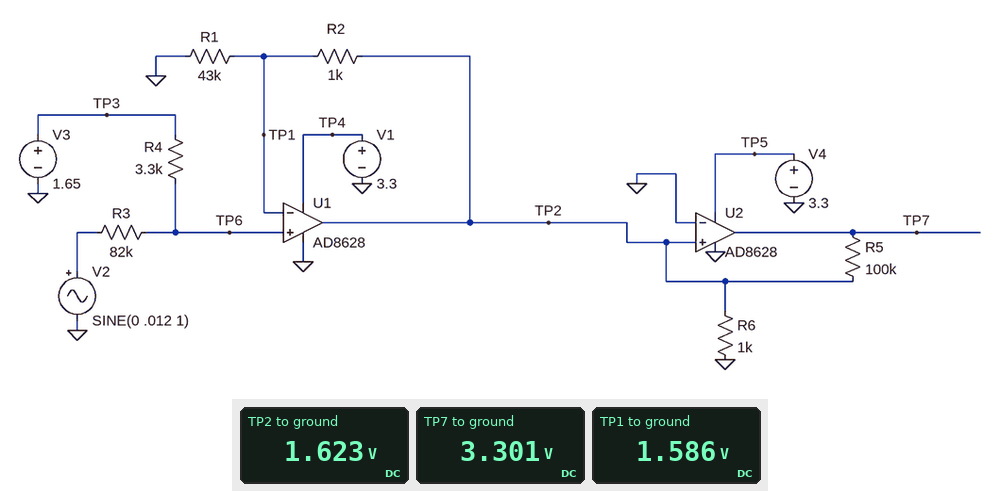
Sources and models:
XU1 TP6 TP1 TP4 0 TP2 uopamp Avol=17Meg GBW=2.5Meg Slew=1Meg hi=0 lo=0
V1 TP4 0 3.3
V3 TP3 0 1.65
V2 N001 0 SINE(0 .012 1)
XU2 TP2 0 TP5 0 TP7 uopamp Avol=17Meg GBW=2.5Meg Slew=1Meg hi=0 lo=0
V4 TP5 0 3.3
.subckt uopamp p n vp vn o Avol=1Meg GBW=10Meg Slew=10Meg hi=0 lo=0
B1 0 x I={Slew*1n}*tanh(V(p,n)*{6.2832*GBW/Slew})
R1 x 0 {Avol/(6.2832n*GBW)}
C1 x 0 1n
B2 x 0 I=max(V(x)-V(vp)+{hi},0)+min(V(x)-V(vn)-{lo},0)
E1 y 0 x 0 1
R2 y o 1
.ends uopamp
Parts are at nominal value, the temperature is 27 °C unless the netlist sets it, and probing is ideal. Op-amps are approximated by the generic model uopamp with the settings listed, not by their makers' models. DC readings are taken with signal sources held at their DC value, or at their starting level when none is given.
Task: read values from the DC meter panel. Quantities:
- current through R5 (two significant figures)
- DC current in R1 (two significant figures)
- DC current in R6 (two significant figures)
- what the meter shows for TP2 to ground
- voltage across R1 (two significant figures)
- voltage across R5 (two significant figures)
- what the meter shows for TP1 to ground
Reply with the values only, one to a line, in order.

17 µA
37 µA
1.6 mA
1.623 V
1.6 V
1.7 V
1.586 V
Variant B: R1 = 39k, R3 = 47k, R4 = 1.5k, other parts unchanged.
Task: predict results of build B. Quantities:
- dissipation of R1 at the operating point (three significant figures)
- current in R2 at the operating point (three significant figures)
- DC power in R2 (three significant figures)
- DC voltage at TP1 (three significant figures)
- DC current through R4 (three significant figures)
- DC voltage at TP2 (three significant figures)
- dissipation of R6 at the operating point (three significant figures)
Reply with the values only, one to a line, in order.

65.6 µW
41.0 µA
1.68 µW
1.60 V
34.0 µA
1.64 V
2.69 mW
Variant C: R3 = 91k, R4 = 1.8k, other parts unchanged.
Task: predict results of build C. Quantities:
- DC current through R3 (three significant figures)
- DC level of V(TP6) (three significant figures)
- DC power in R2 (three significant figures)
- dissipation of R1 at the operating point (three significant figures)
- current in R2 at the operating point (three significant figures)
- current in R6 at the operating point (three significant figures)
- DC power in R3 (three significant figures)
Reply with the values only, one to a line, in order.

17.8 µA
1.62 V
1.42 µW
60.9 µW
37.6 µA
1.66 mA
28.8 µW
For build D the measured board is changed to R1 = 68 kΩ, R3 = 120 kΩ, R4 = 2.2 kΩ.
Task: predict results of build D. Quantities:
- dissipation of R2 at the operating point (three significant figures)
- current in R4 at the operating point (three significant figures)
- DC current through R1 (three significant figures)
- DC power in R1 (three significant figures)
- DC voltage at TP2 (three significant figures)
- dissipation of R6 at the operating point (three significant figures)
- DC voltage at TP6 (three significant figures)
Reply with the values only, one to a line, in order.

568 nW
13.5 µA
23.8 µA
38.6 µW
1.64 V
2.70 mW
1.62 V
